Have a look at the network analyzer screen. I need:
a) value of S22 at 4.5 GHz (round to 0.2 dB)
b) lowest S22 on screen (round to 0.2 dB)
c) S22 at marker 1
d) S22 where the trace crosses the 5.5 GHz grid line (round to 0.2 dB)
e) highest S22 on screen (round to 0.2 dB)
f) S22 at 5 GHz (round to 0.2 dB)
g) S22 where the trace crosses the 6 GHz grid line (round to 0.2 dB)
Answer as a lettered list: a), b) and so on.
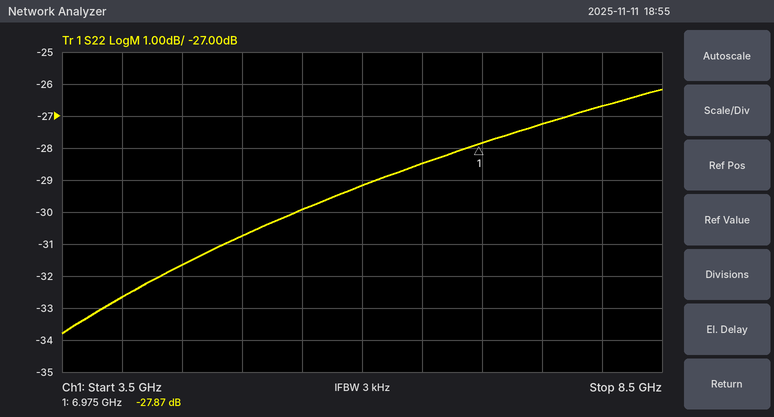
a) -31.6 dB
b) -33.8 dB
c) -27.87 dB
d) -30.0 dB
e) -26.2 dB
f) -30.8 dB
g) -29.2 dB
